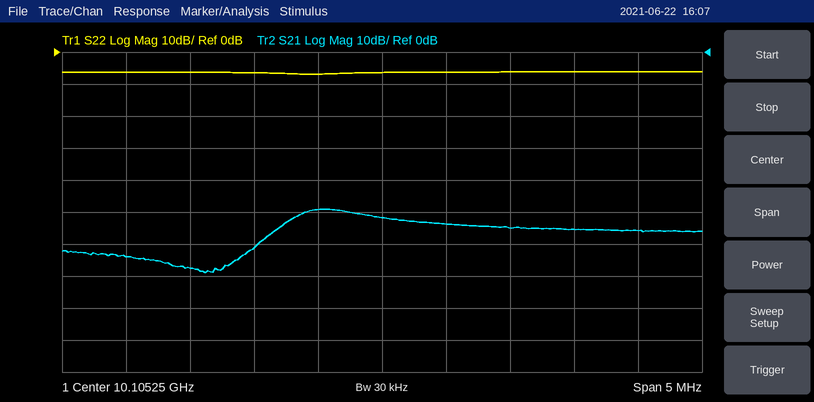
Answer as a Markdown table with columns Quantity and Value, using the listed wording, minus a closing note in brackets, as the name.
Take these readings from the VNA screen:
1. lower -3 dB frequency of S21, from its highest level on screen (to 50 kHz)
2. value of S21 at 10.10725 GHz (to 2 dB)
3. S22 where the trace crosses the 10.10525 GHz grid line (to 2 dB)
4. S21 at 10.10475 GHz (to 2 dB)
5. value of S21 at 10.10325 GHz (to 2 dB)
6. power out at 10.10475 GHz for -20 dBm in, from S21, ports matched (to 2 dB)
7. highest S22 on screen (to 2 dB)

| Quantity | Value |
|---|---|
| lower -3 dB frequency of S21, from its highest level on screen | 10.10455 GHz |
| value of S21 at 10.10725 GHz | -56 dB |
| S22 where the trace crosses the 10.10525 GHz grid line | -6 dB |
| S21 at 10.10475 GHz | -50 dB |
| value of S21 at 10.10325 GHz | -64 dB |
| power out at 10.10475 GHz for -20 dBm in, from S21, ports matched | -70 dBm |
| highest S22 on screen | -6 dB |
